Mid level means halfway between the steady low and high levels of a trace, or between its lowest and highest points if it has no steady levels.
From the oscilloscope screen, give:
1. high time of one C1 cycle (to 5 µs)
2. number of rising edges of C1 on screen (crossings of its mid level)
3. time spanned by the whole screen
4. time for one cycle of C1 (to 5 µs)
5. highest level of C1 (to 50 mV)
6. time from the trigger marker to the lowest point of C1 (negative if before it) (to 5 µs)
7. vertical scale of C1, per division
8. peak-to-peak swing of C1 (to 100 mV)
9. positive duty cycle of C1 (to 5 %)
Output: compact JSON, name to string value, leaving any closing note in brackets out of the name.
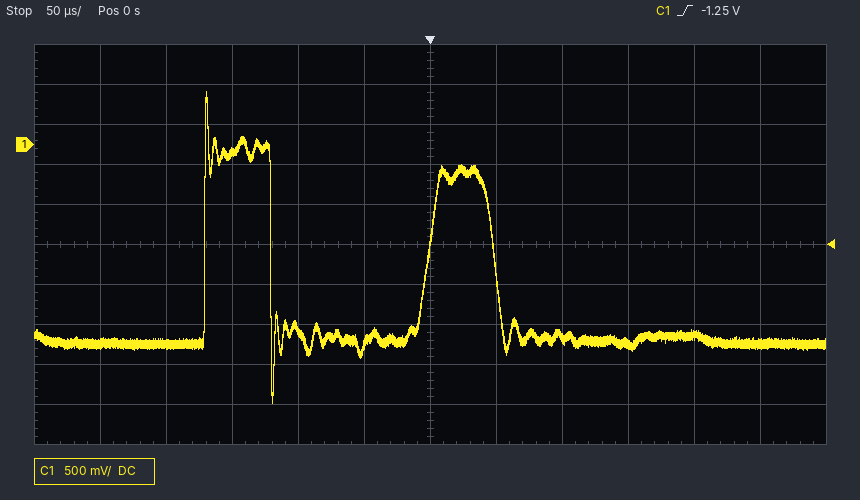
{"high time of one C1 cycle": "50 µs", "number of rising edges of C1 on screen": "2", "time spanned by the whole screen": "600 µs", "time for one cycle of C1": "170 µs", "highest level of C1": "650 mV", "time from the trigger marker to the lowest point of C1 (negative if before it)": "-120 µs", "vertical scale of C1, per division": "500 mV", "peak-to-peak swing of C1": "3.90 V", "positive duty cycle of C1": "30 %"}
